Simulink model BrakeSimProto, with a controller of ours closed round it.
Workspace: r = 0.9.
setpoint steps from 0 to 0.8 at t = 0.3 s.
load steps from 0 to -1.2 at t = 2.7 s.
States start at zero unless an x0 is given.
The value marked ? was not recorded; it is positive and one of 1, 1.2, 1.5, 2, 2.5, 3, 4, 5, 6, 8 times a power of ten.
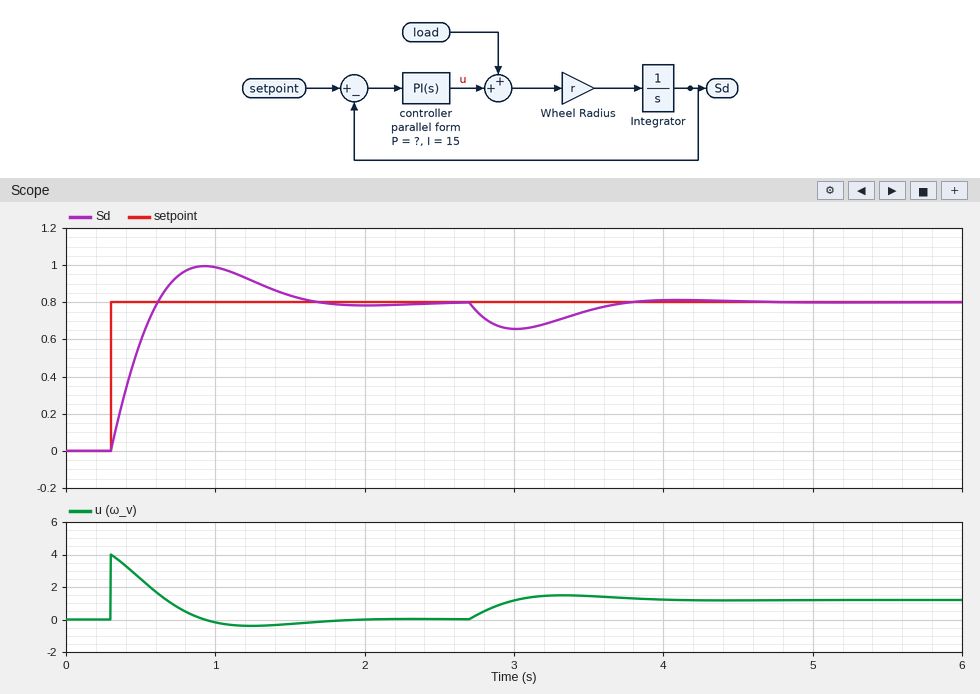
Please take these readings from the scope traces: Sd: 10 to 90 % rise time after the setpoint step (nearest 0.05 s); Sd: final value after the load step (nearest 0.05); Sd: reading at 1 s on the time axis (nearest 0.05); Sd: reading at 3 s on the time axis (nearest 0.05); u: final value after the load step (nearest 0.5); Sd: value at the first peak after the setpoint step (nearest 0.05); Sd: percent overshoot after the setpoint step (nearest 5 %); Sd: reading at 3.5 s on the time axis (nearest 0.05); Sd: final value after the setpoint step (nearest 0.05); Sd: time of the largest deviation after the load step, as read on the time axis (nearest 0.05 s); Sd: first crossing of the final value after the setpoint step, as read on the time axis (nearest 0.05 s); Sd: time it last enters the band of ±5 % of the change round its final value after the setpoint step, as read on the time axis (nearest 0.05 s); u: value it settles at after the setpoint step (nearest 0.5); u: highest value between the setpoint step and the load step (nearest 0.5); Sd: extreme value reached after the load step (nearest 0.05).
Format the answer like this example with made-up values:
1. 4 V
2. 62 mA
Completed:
1. 0.25 s
2. 0.80
3. 1.00
4. 0.65
5. 1.0
6. 1.00
7. 25 %
8. 0.75
9. 0.80
10. 3.00 s
11. 0.60 s
12. 1.50 s
13. 0.0
14. 4.0
15. 0.65
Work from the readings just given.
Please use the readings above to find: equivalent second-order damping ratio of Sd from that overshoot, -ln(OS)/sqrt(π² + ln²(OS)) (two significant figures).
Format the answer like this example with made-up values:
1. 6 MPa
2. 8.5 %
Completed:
1. 0.40
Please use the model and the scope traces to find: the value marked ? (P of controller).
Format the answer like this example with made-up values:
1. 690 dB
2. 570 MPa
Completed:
1. 5
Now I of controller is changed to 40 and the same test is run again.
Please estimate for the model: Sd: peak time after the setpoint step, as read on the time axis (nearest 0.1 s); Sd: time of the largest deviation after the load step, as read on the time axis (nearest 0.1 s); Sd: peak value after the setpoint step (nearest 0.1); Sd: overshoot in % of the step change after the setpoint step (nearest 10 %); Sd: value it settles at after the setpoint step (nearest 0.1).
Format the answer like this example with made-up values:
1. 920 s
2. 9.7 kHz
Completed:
1. 0.7 s
2. 2.9 s
3. 1.1
4. 40 %
5. 0.8
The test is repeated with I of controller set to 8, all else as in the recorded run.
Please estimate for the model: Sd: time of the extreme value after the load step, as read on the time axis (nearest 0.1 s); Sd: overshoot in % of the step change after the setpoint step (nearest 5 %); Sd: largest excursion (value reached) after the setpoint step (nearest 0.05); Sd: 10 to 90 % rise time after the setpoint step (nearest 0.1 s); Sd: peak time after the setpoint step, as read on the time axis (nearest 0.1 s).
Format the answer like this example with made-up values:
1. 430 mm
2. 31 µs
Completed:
1. 3.1 s
2. 15 %
3. 0.95
4. 0.3 s
5. 1.1 s
